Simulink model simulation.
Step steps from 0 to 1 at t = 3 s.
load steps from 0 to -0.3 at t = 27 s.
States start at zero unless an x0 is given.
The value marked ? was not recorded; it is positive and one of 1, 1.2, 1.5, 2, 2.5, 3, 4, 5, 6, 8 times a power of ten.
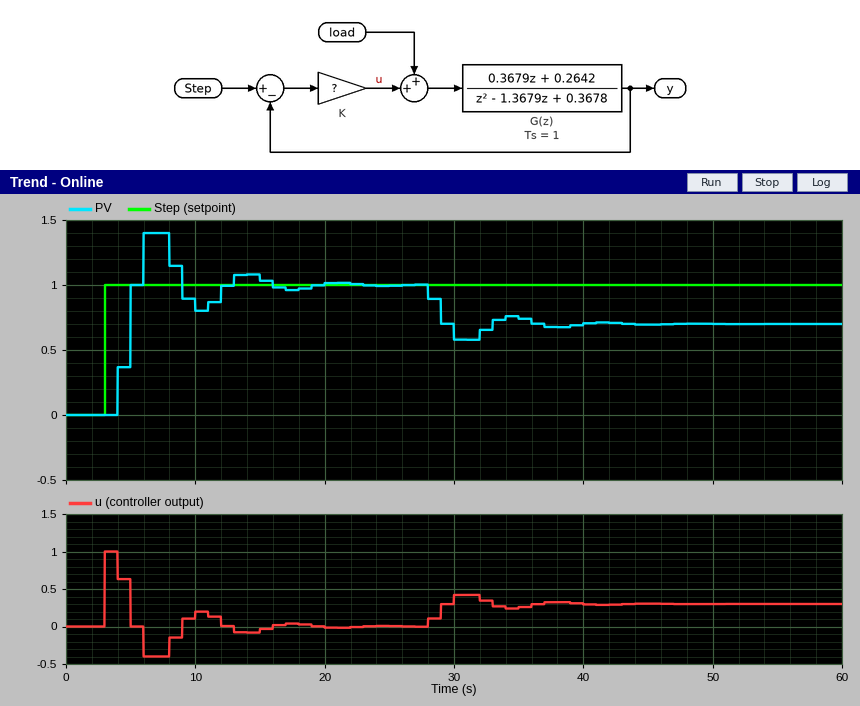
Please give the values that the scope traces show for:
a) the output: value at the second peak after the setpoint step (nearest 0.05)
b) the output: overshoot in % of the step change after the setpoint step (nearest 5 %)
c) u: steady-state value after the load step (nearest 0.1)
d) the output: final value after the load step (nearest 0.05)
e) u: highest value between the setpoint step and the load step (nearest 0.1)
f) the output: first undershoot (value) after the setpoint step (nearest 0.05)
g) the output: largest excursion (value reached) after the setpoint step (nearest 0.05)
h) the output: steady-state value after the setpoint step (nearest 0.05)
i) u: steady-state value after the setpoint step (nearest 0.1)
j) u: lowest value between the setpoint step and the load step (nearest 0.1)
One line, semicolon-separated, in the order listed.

1.10; 40 %; 0.3; 0.70; 1.0; 0.80; 1.40; 1.00; 0.0; -0.4
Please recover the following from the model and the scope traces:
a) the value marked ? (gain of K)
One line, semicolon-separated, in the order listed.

1
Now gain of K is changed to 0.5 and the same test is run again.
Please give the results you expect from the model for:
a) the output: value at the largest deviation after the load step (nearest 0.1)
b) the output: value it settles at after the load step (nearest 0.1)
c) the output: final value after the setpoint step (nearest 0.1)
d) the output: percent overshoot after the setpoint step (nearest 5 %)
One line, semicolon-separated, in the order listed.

0.3; 0.4; 1.0; 15 %
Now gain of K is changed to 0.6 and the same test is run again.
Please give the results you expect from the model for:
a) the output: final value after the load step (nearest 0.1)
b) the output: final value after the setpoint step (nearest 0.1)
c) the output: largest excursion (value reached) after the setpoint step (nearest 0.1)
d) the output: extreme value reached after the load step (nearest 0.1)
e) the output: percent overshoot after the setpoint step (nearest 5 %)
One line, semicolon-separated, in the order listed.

0.5; 1.0; 1.2; 0.4; 20 %
